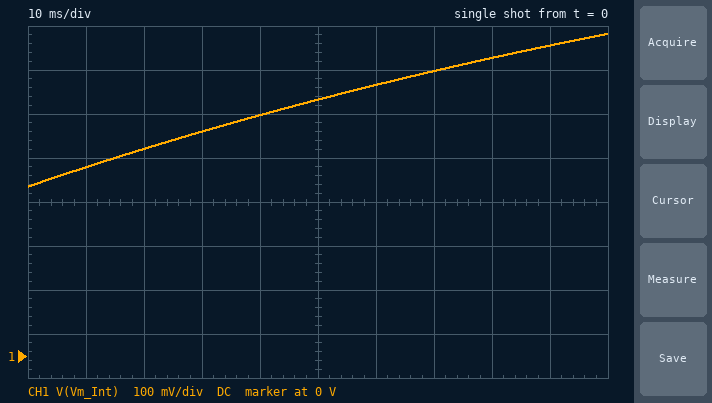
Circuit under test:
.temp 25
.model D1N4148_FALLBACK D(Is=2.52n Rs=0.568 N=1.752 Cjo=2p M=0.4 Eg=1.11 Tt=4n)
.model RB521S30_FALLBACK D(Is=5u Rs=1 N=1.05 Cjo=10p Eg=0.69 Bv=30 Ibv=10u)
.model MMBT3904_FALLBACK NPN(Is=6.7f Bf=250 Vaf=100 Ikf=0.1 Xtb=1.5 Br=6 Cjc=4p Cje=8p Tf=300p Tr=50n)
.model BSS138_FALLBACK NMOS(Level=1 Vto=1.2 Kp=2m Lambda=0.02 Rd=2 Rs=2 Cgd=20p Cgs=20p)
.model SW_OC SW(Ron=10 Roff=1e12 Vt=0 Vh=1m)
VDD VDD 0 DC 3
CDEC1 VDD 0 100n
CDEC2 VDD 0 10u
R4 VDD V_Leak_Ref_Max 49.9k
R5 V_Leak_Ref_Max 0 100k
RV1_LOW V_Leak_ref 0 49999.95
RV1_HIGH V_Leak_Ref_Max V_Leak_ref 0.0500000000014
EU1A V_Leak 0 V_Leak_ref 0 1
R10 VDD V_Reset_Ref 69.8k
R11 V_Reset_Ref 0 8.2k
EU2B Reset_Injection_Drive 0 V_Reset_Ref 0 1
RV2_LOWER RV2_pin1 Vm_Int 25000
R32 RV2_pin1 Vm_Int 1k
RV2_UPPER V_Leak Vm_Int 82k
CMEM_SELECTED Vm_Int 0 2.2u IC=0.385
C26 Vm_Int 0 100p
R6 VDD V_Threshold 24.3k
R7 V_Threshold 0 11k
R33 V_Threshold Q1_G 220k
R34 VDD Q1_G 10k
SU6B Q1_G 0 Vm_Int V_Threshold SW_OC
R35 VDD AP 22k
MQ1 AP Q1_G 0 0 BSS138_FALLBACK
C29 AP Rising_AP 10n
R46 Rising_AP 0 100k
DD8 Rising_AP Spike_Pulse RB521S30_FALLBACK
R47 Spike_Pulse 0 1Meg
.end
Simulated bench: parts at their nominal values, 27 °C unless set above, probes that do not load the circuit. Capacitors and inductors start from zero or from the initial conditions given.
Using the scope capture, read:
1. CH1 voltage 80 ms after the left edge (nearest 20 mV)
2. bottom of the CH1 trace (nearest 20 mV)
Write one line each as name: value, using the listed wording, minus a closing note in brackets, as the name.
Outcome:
CH1 voltage 80 ms after the left edge: 680 mV
bottom of the CH1 trace: 380 mV
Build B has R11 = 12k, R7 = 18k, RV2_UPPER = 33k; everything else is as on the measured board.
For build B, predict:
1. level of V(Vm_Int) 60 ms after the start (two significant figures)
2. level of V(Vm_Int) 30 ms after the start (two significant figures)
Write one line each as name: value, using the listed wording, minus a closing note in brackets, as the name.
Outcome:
level of V(Vm_Int) 60 ms after the start: 840 mV
level of V(Vm_Int) 30 ms after the start: 660 mV
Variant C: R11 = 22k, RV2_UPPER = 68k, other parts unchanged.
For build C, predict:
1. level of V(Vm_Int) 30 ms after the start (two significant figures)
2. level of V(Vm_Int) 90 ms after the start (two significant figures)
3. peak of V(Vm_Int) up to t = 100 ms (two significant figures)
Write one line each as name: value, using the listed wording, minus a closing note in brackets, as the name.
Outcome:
level of V(Vm_Int) 30 ms after the start: 530 mV
level of V(Vm_Int) 90 ms after the start: 750 mV
peak of V(Vm_Int) up to t = 100 ms: 780 mV
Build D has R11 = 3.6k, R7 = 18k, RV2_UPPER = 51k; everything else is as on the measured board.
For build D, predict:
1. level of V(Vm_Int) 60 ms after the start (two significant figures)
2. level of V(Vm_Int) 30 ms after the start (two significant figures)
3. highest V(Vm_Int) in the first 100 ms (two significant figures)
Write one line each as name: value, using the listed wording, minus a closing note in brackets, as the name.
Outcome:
level of V(Vm_Int) 60 ms after the start: 720 mV
level of V(Vm_Int) 30 ms after the start: 580 mV
highest V(Vm_Int) in the first 100 ms: 870 mV
